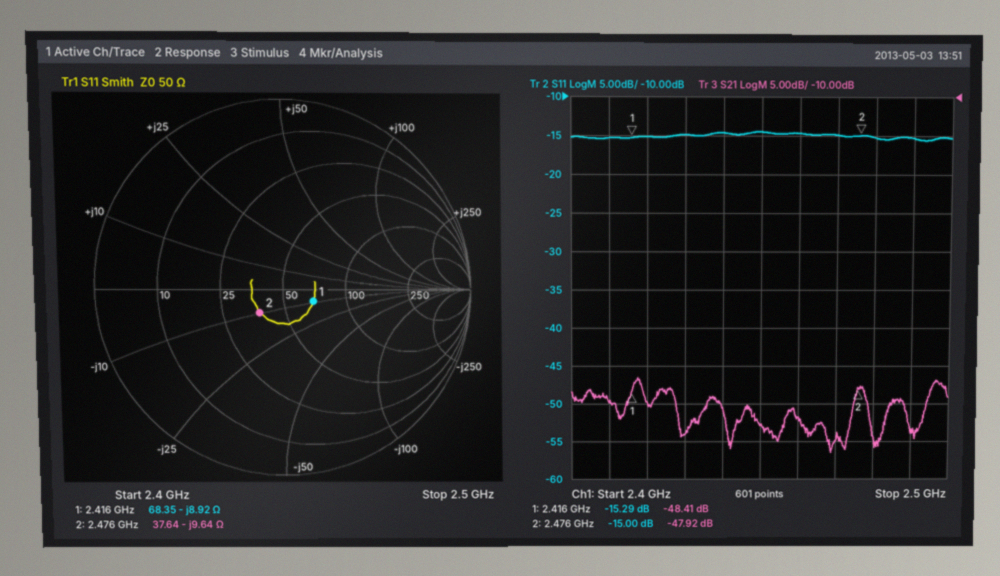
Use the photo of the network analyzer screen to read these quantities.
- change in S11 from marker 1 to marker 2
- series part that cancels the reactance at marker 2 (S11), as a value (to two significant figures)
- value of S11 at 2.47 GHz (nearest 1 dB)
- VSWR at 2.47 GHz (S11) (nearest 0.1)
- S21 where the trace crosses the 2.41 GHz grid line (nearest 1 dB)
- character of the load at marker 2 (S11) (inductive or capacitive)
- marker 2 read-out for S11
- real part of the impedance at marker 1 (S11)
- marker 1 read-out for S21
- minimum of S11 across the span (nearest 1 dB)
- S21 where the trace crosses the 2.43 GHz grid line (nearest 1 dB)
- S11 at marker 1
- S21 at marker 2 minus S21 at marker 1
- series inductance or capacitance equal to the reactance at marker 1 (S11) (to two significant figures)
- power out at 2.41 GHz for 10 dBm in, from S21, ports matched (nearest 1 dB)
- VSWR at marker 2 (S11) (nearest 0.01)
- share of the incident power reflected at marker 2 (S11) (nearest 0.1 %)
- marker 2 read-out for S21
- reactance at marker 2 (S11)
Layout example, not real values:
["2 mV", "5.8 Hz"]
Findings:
["0.29 dB", "620 pH", "-15 dB", "1.4", "-50 dB", "capacitive", "-15.00 dB", "68.35 Ω", "-48.41 dB", "-16 dB", "-54 dB", "-15.29 dB", "0.49 dB", "7.4 pF", "-40 dBm", "1.43", "3.2 %", "-47.92 dB", "-9.64 Ω"]
